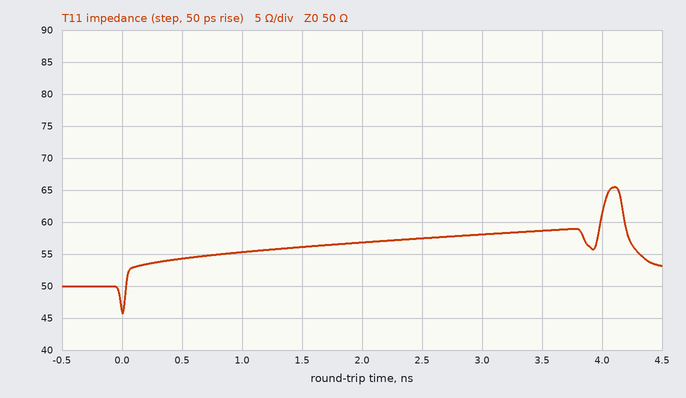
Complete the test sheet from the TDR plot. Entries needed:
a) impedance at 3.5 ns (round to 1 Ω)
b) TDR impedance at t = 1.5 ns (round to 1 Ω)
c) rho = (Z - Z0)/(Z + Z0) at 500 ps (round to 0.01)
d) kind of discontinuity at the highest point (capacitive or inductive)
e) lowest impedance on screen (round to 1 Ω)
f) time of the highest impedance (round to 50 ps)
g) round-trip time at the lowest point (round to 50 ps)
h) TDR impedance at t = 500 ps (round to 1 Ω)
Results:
59 Ω
56 Ω
+0.04
inductive
46 Ω
4.10 ns
0 ps
54 Ω
